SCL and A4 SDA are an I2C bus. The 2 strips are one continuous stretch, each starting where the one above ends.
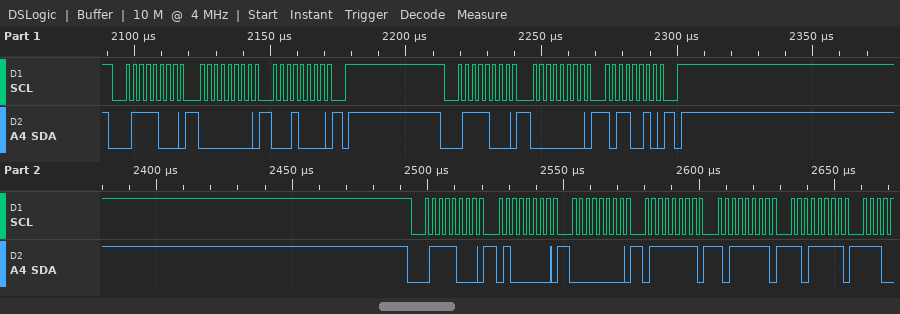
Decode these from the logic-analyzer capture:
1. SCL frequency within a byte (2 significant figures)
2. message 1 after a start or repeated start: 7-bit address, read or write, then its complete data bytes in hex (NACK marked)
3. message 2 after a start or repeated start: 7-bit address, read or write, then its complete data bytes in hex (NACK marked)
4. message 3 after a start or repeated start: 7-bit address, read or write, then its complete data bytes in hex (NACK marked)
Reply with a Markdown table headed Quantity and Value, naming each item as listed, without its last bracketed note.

| Quantity | Value |
|---|---|
| SCL frequency within a byte | 400 kHz |
| message 1 after a start or repeated start: 7-bit address, read or write, then its complete data bytes in hex | 0x3C write: 00 10 |
| message 2 after a start or repeated start: 7-bit address, read or write, then its complete data bytes in hex | 0x3C write: 00 B2 |
| message 3 after a start or repeated start: 7-bit address, read or write, then its complete data bytes in hex | 0x3C write: 40 00 7F BF DF |
